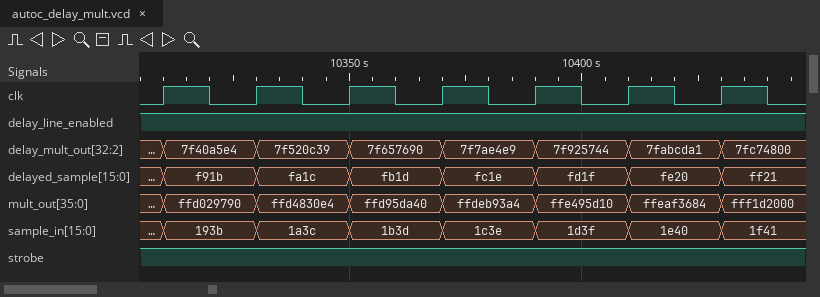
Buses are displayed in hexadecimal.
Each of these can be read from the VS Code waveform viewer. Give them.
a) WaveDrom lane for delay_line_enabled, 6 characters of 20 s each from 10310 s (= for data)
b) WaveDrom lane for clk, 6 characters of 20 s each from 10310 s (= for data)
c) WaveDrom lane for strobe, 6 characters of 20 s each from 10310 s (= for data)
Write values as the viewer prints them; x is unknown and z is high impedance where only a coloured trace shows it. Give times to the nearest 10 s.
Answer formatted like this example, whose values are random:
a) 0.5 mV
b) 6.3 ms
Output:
a) {name: 'delay_line_enabled', wave: '1.....'}
b) {name: 'clk', wave: 'p.....'}
c) {name: 'strobe', wave: '1.....'}
